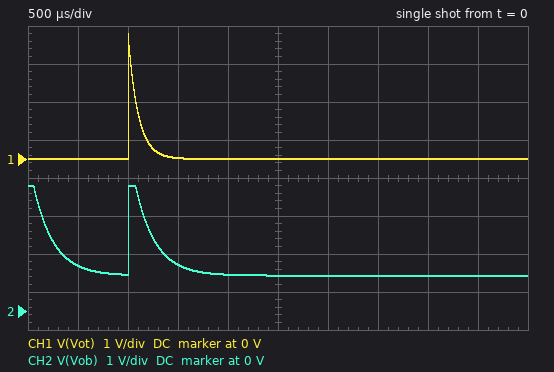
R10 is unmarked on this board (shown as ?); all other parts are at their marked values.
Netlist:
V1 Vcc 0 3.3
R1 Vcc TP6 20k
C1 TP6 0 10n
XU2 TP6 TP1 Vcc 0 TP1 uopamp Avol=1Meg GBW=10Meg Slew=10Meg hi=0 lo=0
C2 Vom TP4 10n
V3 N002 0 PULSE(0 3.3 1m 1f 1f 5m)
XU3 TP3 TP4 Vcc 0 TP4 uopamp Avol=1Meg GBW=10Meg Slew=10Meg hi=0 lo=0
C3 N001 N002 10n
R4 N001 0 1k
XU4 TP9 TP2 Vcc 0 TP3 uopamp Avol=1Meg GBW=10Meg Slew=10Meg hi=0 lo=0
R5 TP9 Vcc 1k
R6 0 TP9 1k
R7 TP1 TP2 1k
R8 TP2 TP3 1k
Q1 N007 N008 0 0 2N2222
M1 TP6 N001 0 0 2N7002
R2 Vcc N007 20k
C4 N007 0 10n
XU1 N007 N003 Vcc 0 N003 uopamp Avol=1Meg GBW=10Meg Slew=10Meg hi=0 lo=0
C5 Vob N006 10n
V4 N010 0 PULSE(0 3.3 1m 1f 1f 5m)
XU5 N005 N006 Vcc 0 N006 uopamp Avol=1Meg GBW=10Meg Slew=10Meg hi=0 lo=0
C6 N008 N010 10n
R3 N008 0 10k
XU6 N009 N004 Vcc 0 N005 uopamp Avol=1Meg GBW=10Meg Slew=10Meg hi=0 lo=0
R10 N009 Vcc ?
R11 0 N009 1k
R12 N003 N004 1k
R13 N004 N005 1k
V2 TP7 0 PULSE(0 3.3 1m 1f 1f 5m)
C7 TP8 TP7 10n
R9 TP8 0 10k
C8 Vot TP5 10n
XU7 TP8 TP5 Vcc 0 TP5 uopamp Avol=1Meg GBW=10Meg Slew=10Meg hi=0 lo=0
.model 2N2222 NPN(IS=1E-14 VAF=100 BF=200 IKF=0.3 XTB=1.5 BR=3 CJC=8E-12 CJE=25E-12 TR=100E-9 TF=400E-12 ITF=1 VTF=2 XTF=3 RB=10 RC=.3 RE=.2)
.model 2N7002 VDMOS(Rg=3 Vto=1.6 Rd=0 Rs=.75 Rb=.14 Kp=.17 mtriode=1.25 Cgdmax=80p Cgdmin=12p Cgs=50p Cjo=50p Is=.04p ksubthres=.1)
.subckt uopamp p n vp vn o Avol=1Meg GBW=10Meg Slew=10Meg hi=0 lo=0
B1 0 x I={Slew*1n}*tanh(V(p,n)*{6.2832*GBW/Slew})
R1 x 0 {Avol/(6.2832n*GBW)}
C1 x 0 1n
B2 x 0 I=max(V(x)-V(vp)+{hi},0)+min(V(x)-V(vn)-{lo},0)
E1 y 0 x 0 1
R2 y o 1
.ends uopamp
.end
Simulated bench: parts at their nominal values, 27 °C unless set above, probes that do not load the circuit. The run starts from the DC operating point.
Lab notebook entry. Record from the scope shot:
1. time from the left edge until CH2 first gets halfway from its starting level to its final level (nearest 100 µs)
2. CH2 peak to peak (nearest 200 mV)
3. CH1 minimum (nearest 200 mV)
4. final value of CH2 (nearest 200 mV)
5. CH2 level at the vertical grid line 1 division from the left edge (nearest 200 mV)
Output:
200 µs
2.4 V
0 V
1.0 V
1.2 V
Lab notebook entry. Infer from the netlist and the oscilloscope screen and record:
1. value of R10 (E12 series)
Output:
560 Ω
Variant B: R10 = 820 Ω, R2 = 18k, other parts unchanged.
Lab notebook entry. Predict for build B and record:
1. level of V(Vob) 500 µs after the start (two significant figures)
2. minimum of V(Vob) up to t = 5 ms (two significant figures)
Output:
520 mV
330 mV
